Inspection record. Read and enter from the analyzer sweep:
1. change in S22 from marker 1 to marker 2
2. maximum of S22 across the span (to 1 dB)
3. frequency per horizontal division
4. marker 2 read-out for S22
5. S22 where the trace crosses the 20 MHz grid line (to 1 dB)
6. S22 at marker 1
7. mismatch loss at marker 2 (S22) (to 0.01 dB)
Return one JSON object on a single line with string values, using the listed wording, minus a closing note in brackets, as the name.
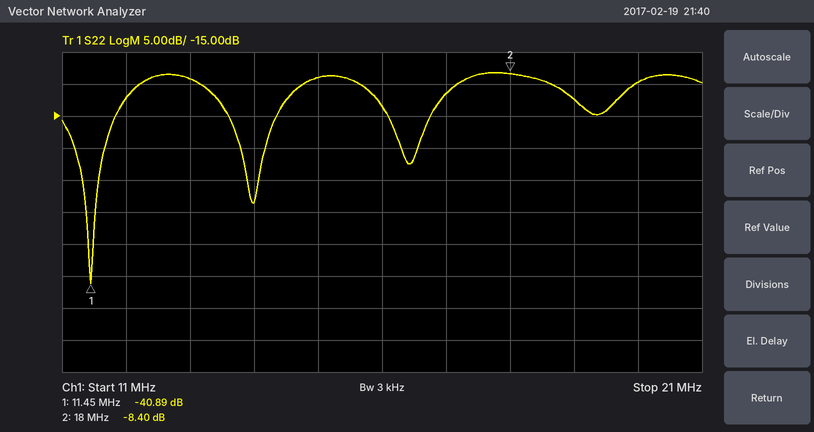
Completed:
{"change in S22 from marker 1 to marker 2": "32.49 dB", "maximum of S22 across the span": "-8 dB", "frequency per horizontal division": "1 MHz", "marker 2 read-out for S22": "-8.40 dB", "S22 where the trace crosses the 20 MHz grid line": "-10 dB", "S22 at marker 1": "-40.89 dB", "mismatch loss at marker 2 (S22)": "0.68 dB"}
